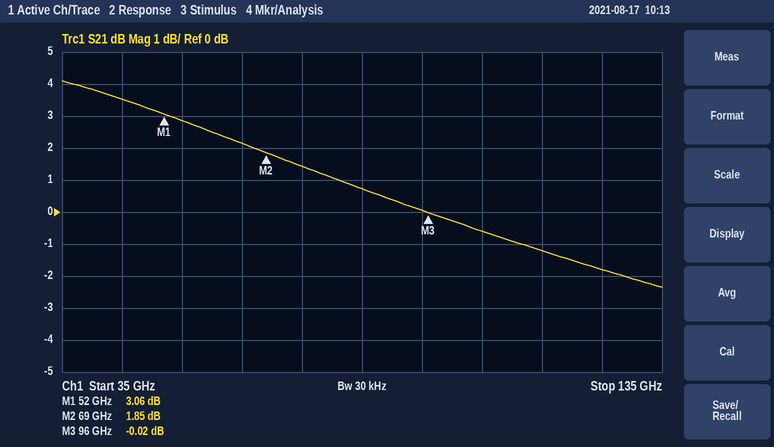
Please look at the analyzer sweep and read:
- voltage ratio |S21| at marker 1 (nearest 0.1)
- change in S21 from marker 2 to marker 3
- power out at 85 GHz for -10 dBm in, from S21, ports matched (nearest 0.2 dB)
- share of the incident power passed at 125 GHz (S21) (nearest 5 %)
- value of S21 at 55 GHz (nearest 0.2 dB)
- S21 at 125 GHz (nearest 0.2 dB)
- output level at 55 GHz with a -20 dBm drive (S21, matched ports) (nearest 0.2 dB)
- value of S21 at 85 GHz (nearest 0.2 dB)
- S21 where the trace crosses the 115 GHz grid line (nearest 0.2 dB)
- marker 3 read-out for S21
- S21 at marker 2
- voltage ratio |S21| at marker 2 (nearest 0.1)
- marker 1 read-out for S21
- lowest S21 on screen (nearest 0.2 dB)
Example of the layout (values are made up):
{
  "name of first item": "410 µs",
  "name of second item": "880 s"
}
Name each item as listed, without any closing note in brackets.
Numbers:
{
  "voltage ratio |S21| at marker 1": "1.4",
  "change in S21 from marker 2 to marker 3": "-1.87 dB",
  "power out at 85 GHz for -10 dBm in, from S21, ports matched": "-9.2 dBm",
  "share of the incident power passed at 125 GHz (S21)": "65 %",
  "value of S21 at 55 GHz": "2.8 dB",
  "S21 at 125 GHz": "-1.8 dB",
  "output level at 55 GHz with a -20 dBm drive (S21, matched ports)": "-17.2 dBm",
  "value of S21 at 85 GHz": "0.8 dB",
  "S21 where the trace crosses the 115 GHz grid line": "-1.2 dB",
  "marker 3 read-out for S21": "-0.02 dB",
  "S21 at marker 2": "1.85 dB",
  "voltage ratio |S21| at marker 2": "1.2",
  "marker 1 read-out for S21": "3.06 dB",
  "lowest S21 on screen": "-2.4 dB"
}
